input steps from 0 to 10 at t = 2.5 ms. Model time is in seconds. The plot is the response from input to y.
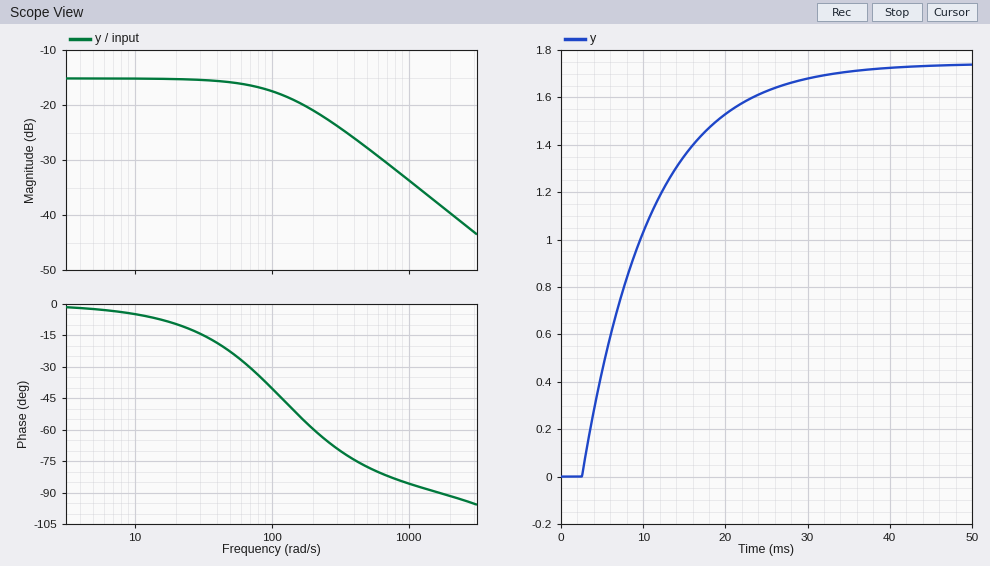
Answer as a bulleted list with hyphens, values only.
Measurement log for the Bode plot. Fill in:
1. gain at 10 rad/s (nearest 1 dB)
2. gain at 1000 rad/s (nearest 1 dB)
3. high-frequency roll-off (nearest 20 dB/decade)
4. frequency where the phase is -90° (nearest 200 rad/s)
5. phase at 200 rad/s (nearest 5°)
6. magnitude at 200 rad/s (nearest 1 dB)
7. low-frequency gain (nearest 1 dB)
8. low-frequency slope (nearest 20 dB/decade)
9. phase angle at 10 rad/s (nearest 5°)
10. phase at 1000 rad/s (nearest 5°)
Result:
- -15 dB
- -34 dB
- -20 dB/decade
- 1600 rad/s
- -60°
- -21 dB
- -15 dB
- 0 dB/decade
- -5°
- -85°
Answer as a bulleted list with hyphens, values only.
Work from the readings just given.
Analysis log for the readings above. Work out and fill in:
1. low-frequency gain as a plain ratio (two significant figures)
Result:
- 0.18
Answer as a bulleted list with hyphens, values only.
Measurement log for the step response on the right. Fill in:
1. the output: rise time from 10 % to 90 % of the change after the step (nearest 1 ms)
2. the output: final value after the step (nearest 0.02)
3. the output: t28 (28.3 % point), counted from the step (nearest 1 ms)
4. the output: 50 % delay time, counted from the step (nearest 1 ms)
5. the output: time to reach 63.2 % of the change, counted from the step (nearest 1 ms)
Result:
- 18 ms
- 1.74
- 3 ms
- 6 ms
- 8 ms
